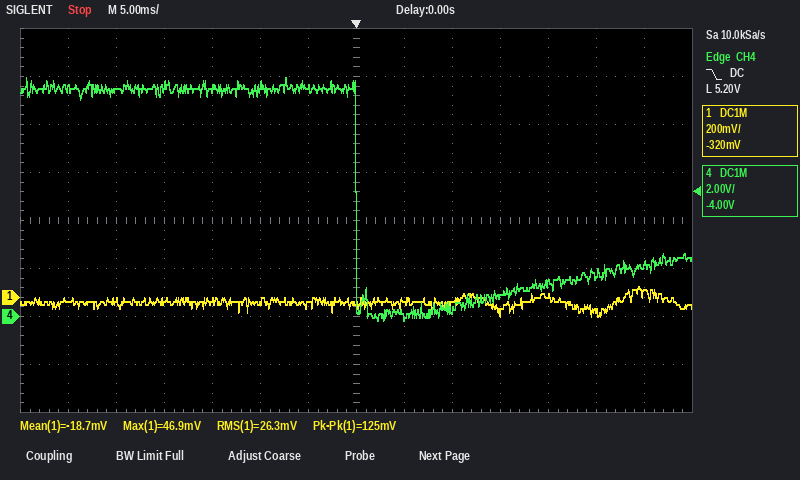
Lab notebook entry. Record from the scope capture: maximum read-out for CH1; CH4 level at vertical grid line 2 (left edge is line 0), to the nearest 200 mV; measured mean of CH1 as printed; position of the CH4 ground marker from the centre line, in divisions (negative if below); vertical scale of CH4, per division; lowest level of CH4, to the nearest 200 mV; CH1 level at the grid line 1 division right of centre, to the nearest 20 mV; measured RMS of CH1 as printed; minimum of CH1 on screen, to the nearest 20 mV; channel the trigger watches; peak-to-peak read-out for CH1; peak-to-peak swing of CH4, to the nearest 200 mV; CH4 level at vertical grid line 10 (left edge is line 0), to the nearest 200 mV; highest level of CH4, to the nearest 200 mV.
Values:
46.9 mV
9.4 V
-18.7 mV
-2.0 div
2 V
-200 mV
-20 mV
26.3 mV
-80 mV
CH4
125 mV
10.2 V
800 mV
10.0 V
